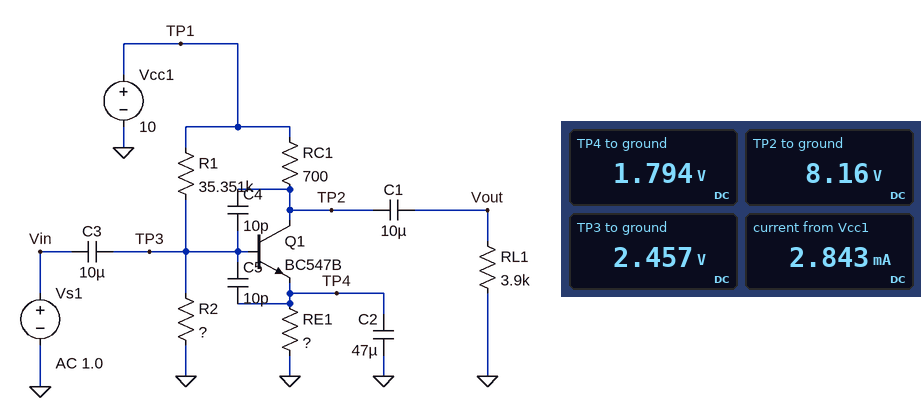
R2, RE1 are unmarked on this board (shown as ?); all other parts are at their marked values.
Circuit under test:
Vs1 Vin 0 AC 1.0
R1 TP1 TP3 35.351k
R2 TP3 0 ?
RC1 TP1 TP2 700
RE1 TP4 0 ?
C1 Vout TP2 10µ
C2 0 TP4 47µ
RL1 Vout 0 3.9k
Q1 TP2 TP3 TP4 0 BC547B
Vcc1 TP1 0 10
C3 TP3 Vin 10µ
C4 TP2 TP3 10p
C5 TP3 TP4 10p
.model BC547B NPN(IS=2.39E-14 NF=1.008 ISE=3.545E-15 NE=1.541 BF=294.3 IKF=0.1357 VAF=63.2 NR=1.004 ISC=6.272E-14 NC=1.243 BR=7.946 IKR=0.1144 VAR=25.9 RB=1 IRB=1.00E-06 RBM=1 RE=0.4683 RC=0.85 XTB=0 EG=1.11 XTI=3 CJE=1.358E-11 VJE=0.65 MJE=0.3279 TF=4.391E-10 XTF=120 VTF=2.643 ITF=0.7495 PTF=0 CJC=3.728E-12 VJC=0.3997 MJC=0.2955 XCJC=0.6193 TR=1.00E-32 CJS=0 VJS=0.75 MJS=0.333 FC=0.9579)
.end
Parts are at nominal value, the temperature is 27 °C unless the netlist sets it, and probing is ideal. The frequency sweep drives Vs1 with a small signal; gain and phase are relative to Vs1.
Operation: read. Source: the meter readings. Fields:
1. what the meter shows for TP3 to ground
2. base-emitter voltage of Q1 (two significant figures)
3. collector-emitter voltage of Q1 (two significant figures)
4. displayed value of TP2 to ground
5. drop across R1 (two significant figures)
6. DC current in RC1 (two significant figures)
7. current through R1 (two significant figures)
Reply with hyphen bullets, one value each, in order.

- 2.457 V
- 660 mV
- 6.4 V
- 8.16 V
- 7.5 V
- 2.6 mA
- 210 µA
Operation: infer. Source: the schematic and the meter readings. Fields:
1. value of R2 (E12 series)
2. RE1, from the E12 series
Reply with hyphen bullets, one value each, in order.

- 12 kΩ
- 680 Ω
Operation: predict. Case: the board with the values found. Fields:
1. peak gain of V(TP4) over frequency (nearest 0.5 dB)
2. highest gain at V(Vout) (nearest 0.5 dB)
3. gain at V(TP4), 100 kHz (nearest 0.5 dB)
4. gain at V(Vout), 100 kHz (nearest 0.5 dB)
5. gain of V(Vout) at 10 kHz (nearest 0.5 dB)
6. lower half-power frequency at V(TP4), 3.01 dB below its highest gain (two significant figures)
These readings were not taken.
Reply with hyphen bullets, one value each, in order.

- -0.5 dB
- 35.0 dB
- -50.0 dB
- 35.0 dB
- 35.0 dB
- 1.8 Hz
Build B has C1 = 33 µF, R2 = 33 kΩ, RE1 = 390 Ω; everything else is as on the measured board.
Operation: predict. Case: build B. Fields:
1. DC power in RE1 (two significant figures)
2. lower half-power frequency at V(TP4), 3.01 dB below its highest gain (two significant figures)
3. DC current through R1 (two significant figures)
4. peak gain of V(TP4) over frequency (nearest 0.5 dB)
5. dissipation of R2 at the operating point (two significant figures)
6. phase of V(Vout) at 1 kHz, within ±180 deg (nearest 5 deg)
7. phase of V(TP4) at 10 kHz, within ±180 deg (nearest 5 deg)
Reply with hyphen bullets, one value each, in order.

- 32 mW
- 3.0 Hz
- 160 µA
- -1.5 dB
- 540 µW
- -140 deg
- -85 deg
